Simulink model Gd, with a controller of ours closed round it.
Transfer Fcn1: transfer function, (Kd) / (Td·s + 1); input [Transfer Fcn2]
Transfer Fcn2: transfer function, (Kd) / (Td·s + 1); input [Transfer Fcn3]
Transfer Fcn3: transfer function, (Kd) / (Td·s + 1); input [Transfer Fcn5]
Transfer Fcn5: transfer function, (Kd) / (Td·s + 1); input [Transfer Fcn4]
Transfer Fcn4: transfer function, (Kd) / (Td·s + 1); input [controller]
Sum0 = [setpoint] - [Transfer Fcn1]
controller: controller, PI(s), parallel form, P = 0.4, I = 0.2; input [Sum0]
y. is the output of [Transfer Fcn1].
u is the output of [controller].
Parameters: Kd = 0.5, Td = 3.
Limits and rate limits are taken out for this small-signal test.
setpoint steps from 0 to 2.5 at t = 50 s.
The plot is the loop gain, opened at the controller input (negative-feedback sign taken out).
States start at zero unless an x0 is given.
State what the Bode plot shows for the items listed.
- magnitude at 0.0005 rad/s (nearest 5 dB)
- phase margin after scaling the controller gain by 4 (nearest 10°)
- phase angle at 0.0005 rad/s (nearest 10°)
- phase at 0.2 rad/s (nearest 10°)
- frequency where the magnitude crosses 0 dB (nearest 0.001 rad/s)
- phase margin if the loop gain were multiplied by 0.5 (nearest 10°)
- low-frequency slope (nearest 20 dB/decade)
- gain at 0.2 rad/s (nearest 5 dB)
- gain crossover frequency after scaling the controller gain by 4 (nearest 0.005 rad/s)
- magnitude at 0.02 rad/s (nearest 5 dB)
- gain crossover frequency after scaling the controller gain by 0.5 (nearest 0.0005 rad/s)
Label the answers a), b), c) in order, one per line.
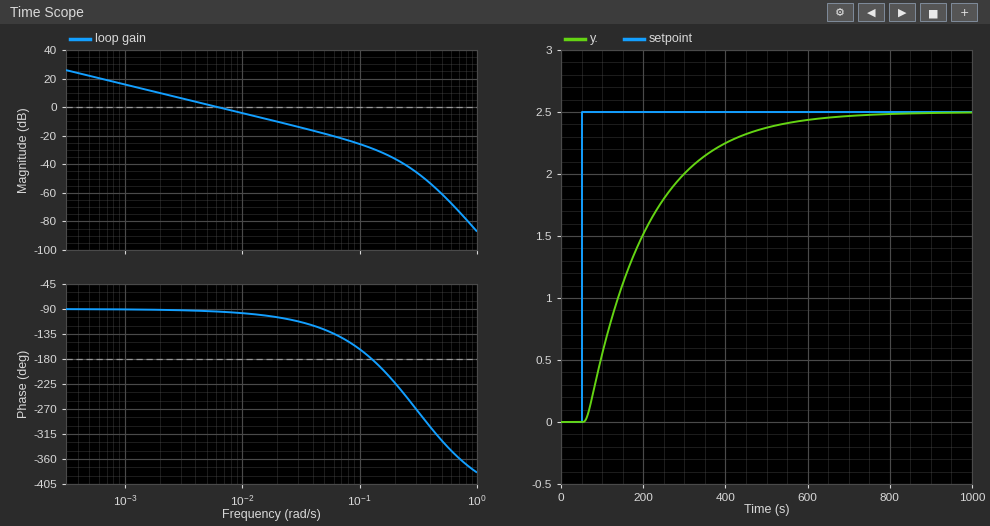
a) 20 dB
b) 70°
c) -90°
d) -220°
e) 0.006 rad/s
f) 90°
g) -20 dB/decade
h) -35 dB
i) 0.025 rad/s
j) -10 dB
k) 0.0030 rad/s
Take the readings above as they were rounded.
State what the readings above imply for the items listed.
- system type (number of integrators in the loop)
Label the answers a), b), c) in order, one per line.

a) 1
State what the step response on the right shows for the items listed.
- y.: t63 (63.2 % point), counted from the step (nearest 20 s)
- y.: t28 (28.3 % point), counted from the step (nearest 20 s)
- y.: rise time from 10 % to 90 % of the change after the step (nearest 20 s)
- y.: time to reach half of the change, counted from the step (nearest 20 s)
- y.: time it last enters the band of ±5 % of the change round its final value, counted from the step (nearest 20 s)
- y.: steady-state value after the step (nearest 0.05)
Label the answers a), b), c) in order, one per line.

a) 160 s
b) 60 s
c) 320 s
d) 120 s
e) 460 s
f) 2.50
